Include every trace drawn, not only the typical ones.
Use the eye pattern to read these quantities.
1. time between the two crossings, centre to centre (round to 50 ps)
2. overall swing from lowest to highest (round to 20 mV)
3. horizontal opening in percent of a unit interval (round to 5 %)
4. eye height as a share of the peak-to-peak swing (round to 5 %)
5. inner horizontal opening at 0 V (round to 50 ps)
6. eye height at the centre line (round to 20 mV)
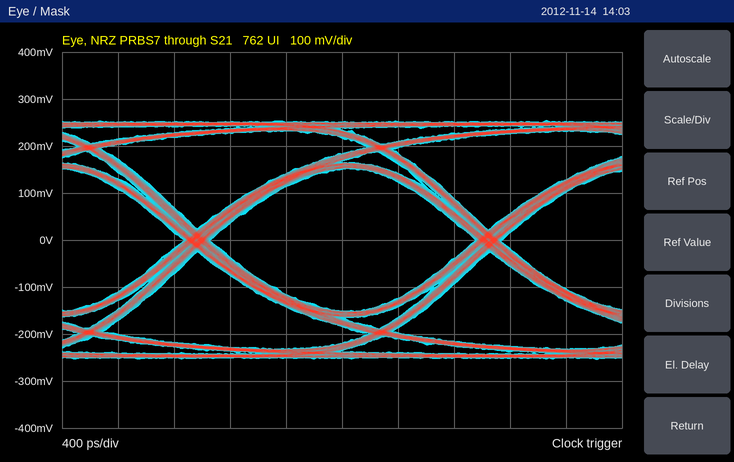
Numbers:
2.10 ns
500 mV
90 %
60 %
1.90 ns
300 mV
